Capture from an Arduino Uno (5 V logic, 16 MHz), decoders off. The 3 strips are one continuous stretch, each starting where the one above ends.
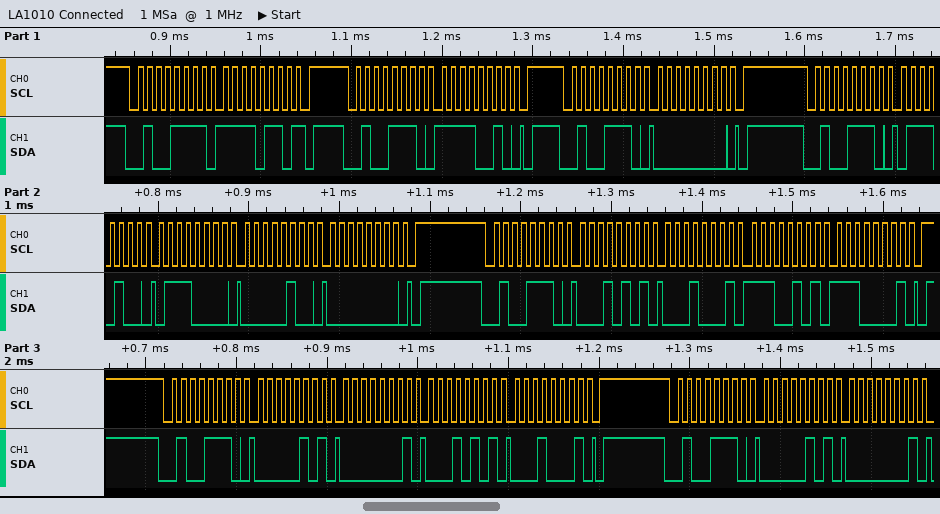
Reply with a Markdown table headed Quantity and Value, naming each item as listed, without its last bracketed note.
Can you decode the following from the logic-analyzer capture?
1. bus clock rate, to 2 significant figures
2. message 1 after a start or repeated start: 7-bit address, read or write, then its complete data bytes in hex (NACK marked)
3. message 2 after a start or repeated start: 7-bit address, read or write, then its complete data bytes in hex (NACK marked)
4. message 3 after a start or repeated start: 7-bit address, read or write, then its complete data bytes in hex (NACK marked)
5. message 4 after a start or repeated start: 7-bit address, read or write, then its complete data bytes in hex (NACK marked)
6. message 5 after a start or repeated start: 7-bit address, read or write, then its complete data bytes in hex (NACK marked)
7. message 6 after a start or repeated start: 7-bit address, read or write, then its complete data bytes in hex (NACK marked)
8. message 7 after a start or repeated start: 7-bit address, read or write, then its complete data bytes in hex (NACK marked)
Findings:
| Quantity | Value |
|---|---|
| bus clock rate, to 2 significant figures | 100 kHz |
| message 1 after a start or repeated start: 7-bit address, read or write, then its complete data bytes in hex | 0x27 read: F6 NACK |
| message 2 after a start or repeated start: 7-bit address, read or write, then its complete data bytes in hex | 0x27 write: F2 |
| message 3 after a start or repeated start: 7-bit address, read or write, then its complete data bytes in hex | 0x27 write: 00 |
| message 4 after a start or repeated start: 7-bit address, read or write, then its complete data bytes in hex | 0x27 write: 74 70 04 00 |
| message 5 after a start or repeated start: 7-bit address, read or write, then its complete data bytes in hex | 0x27 write: 15 11 E5 E1 |
| message 6 after a start or repeated start: 7-bit address, read or write, then its complete data bytes in hex | 0x27 write: 05 01 15 11 |
| message 7 after a start or repeated start: 7-bit address, read or write, then its complete data bytes in hex | 0x27 write: 05 01 |
